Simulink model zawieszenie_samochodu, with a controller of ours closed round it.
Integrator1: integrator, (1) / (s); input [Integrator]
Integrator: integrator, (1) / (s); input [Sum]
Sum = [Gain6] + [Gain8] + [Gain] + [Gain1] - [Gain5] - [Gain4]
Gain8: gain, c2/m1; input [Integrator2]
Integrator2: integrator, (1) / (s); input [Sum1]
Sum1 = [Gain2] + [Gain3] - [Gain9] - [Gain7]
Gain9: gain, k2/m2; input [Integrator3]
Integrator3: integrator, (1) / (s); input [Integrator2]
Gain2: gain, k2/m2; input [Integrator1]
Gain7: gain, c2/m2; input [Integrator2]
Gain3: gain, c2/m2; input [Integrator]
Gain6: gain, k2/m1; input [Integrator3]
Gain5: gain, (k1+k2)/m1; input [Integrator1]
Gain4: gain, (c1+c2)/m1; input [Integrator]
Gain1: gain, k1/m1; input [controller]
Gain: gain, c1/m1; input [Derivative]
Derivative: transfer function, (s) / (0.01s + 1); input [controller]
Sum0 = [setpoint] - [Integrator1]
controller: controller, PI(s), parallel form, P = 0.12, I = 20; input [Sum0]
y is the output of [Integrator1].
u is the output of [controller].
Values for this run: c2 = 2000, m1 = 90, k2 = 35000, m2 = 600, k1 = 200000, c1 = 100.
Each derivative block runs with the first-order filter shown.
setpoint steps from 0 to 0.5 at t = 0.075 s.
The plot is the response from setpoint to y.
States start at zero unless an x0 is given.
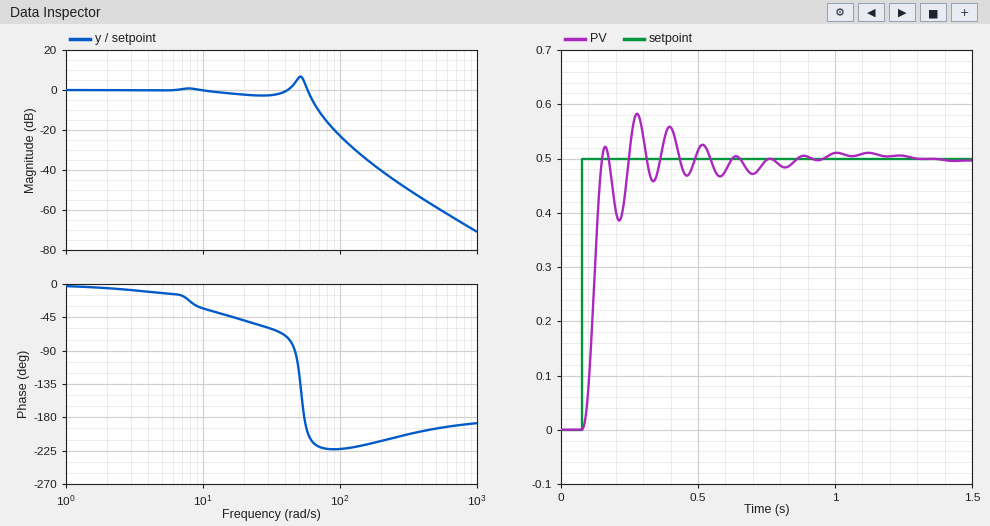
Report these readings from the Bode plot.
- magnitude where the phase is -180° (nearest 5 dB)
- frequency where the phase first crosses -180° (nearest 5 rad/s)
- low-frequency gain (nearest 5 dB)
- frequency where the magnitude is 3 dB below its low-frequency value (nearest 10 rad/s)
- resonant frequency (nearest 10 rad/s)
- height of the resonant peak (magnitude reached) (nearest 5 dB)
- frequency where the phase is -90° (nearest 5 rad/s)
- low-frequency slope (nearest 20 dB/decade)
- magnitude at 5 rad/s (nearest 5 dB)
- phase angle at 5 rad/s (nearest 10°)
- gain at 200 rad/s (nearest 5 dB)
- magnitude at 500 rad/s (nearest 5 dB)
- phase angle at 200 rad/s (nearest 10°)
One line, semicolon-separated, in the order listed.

5 dB; 55 rad/s; 0 dB; 60 rad/s; 50 rad/s; 5 dB; 45 rad/s; 0 dB/decade; 0 dB; -10°; -40 dB; -60 dB; -210°
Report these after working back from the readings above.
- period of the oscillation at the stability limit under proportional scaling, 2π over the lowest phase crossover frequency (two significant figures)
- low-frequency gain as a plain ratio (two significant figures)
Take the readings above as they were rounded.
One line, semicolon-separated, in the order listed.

0.11 s; 1.0
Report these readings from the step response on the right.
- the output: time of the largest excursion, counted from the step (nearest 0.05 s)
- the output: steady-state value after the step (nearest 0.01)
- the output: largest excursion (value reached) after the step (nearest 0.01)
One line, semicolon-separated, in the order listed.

0.20 s; 0.50; 0.58
